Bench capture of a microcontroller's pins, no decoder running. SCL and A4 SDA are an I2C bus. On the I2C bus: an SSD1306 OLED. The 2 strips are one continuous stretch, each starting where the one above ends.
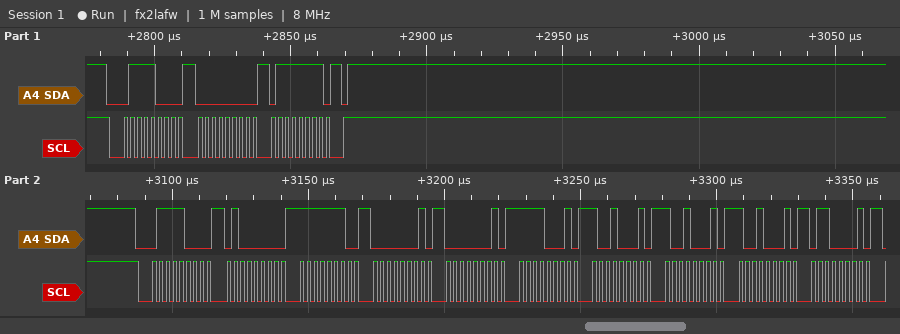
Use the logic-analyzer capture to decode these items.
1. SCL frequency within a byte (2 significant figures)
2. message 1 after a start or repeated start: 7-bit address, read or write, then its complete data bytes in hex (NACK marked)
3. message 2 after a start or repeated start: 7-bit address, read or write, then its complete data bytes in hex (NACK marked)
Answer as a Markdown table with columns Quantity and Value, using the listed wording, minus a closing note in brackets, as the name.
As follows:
| Quantity | Value |
|---|---|
| SCL frequency within a byte | 400 kHz |
| message 1 after a start or repeated start: 7-bit address, read or write, then its complete data bytes in hex | 0x3C write: 00 7F |
| message 2 after a start or repeated start: 7-bit address, read or write, then its complete data bytes in hex | 0x3C write: 40 FE 01 01 F1 91 91 91 61 |
